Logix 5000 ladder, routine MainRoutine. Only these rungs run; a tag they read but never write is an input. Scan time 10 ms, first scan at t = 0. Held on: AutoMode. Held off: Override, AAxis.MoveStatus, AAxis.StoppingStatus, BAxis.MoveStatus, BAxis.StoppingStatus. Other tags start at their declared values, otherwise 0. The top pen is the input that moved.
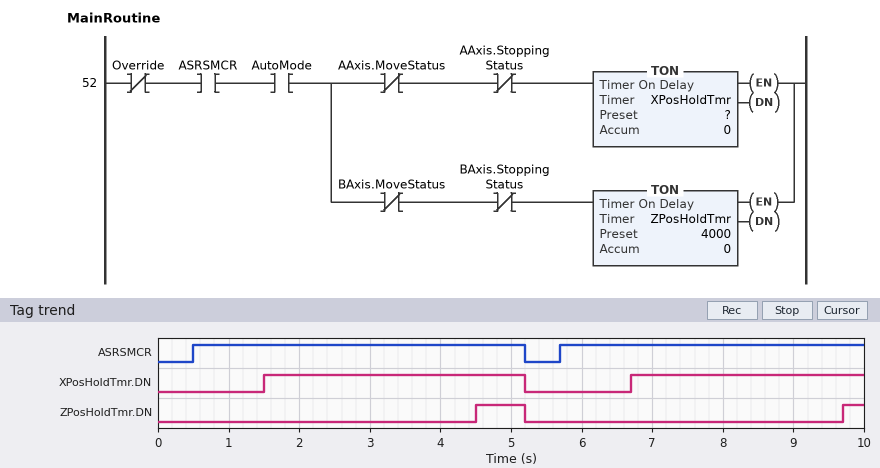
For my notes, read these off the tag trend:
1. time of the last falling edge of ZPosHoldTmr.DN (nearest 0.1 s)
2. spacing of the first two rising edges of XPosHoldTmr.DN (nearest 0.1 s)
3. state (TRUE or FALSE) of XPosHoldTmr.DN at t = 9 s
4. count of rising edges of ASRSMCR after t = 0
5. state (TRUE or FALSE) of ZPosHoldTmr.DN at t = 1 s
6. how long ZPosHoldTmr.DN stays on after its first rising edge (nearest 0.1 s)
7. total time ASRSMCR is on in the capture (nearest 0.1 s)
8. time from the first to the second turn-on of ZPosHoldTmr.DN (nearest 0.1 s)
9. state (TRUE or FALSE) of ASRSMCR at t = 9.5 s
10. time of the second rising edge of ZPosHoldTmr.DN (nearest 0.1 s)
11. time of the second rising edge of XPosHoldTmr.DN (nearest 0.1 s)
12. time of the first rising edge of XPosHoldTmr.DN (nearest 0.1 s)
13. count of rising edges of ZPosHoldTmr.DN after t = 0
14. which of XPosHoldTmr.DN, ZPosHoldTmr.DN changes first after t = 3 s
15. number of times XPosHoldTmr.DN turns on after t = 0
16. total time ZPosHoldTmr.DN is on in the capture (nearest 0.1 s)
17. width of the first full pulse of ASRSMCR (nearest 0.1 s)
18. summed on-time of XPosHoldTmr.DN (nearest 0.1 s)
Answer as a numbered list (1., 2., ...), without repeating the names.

1. 5.2 s
2. 5.2 s
3. TRUE
4. 2
5. FALSE
6. 0.7 s
7. 9.0 s
8. 5.2 s
9. TRUE
10. 9.7 s
11. 6.7 s
12. 1.5 s
13. 2
14. ZPosHoldTmr.DN
15. 2
16. 1.0 s
17. 4.7 s
18. 7.0 s
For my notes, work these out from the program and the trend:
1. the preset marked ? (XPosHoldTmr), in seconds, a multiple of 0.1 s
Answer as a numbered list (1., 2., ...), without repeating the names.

1. 1.0 s
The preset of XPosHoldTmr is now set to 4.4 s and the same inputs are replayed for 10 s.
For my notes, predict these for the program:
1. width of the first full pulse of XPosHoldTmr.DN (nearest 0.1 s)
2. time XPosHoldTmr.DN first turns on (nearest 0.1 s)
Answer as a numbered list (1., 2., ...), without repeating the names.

1. 0.3 s
2. 4.9 s
